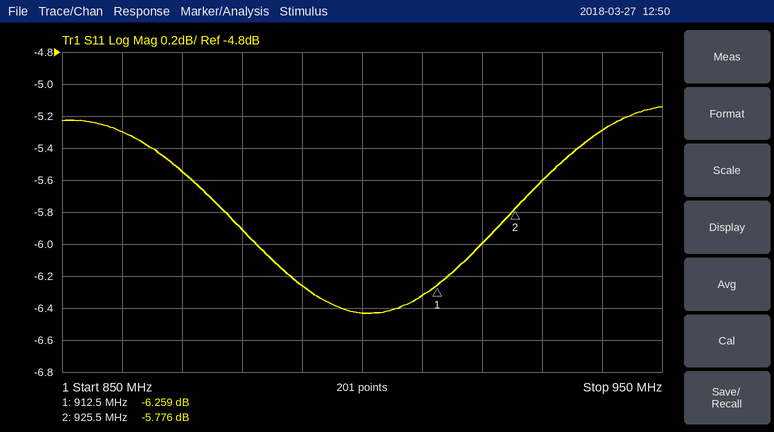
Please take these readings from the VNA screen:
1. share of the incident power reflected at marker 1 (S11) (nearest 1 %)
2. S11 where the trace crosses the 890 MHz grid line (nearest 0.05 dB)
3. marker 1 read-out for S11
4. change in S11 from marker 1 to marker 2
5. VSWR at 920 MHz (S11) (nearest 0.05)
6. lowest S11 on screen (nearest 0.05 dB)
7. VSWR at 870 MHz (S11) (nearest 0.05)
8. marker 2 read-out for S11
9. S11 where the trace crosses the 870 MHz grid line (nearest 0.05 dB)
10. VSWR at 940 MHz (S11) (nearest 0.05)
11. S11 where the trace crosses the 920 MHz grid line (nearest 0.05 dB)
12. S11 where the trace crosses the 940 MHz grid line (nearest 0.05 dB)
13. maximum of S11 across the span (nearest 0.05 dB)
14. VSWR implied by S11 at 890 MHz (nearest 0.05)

24 %
-6.25 dB
-6.259 dB
0.483 dB
3.00
-6.45 dB
3.25
-5.776 dB
-5.55 dB
3.40
-6.00 dB
-5.30 dB
-5.15 dB
2.90
